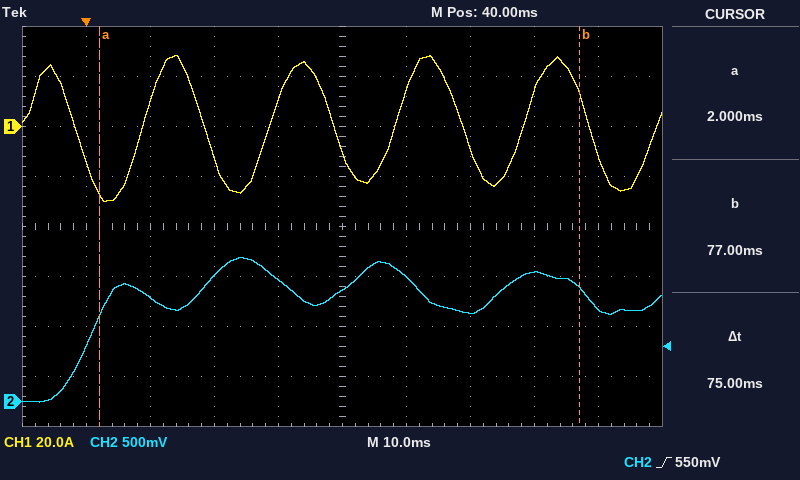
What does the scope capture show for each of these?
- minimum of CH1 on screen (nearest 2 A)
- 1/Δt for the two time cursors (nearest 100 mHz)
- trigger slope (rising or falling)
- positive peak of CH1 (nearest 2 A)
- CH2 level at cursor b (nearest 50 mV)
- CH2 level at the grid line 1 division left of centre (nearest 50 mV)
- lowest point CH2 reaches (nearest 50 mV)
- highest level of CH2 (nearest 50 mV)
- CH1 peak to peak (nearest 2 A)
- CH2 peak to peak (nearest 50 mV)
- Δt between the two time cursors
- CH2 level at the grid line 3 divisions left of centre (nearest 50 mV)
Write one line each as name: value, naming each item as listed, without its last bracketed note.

minimum of CH1 on screen: -30 A
1/Δt for the two time cursors: 13.3 Hz
trigger slope: rising
positive peak of CH1: 28 A
CH2 level at cursor b: 1.15 V
CH2 level at the grid line 1 division left of centre: 1.20 V
lowest point CH2 reaches: 0 mV
highest level of CH2: 1.45 V
CH1 peak to peak: 58 A
CH2 peak to peak: 1.45 V
Δt between the two time cursors: 75 ms
CH2 level at the grid line 3 divisions left of centre: 1.05 V
